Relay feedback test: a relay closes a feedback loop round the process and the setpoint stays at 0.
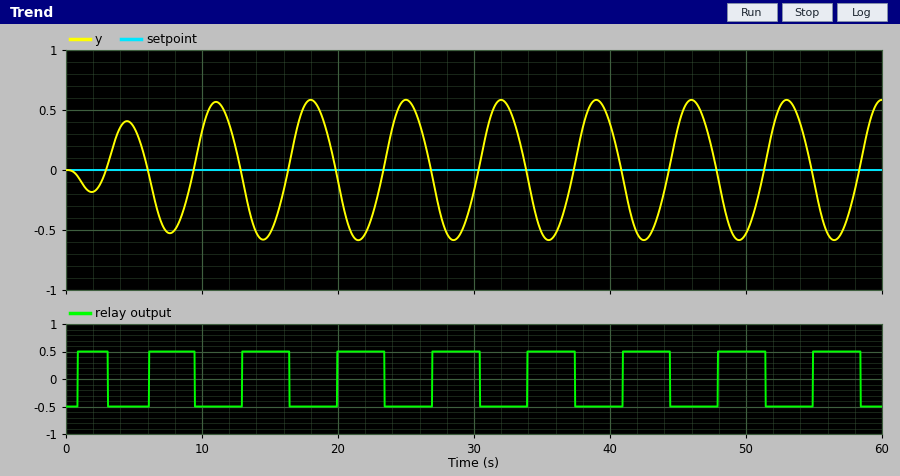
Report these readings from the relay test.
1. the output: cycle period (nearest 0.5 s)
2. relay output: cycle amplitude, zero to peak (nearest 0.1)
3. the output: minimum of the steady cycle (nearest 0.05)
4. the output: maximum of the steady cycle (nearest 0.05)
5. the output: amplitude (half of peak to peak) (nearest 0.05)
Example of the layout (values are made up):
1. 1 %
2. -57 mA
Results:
1. 7.0 s
2. 0.5
3. -0.60
4. 0.60
5. 0.60
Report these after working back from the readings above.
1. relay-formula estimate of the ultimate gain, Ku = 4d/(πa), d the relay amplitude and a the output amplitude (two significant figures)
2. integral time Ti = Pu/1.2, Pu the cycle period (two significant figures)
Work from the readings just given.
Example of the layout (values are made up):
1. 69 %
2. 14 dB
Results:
1. 1.1
2. 5.8 s
